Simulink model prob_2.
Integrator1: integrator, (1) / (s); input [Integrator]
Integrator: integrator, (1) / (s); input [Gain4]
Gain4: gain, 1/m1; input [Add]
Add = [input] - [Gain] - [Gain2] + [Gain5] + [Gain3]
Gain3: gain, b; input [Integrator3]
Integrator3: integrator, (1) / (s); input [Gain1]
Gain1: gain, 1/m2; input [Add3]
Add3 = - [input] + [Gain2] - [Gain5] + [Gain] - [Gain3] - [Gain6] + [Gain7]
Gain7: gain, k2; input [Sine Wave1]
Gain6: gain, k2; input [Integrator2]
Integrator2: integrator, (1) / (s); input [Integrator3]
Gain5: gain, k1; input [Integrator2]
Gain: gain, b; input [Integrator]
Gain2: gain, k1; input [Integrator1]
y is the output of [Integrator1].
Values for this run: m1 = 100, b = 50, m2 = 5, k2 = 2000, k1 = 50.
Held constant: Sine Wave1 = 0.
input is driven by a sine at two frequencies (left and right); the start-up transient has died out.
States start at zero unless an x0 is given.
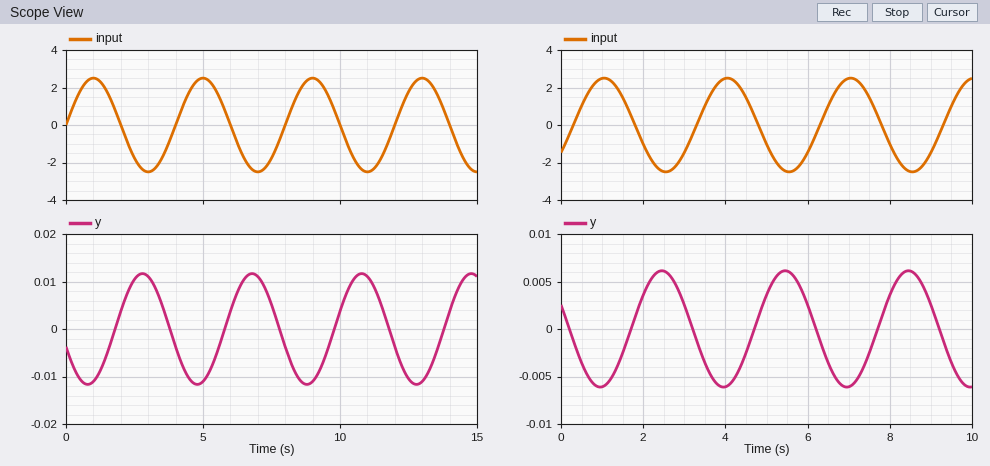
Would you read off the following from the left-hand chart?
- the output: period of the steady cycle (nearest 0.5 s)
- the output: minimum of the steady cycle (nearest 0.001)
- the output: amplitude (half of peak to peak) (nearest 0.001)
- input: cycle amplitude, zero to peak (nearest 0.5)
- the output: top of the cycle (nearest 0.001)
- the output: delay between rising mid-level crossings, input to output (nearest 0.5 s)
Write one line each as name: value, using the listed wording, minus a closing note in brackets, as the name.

the output: period of the steady cycle: 4.0 s
the output: minimum of the steady cycle: -0.012
the output: amplitude (half of peak to peak): 0.012
input: cycle amplitude, zero to peak: 2.5
the output: top of the cycle: 0.012
the output: delay between rising mid-level crossings, input to output: 2.0 s
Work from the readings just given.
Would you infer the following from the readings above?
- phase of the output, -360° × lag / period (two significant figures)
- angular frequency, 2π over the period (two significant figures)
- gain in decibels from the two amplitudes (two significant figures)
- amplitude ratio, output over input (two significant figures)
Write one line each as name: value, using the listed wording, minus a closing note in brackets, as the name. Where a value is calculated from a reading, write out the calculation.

phase of the output, -360° × lag / period: -360 × 2 / 4 = -180°
angular frequency, 2π over the period: 2π / 4 = 1.6 rad/s
gain in decibels from the two amplitudes: 20 log10(0.012 / 2.5) = -46 dB
amplitude ratio, output over input: 0.012 / 2.5 = 0.0048
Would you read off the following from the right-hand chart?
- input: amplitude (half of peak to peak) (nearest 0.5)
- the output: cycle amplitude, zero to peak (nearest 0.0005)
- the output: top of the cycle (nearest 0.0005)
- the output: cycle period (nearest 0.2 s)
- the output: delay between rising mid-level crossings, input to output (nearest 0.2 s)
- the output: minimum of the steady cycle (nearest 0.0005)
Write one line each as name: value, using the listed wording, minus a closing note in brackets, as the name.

input: amplitude (half of peak to peak): 2.5
the output: cycle amplitude, zero to peak: 0.0060
the output: top of the cycle: 0.0060
the output: cycle period: 3.0 s
the output: delay between rising mid-level crossings, input to output: 1.4 s
the output: minimum of the steady cycle: -0.0060
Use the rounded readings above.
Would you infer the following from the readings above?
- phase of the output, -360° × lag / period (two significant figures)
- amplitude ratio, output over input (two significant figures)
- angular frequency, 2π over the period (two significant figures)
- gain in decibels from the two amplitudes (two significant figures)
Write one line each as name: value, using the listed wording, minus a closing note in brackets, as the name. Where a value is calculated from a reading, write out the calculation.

phase of the output, -360° × lag / period: -360 × 1.4 / 3 = -170°
amplitude ratio, output over input: 0.006 / 2.5 = 0.0024
angular frequency, 2π over the period: 2π / 3 = 2.1 rad/s
gain in decibels from the two amplitudes: 20 log10(0.006 / 2.5) = -52 dB
